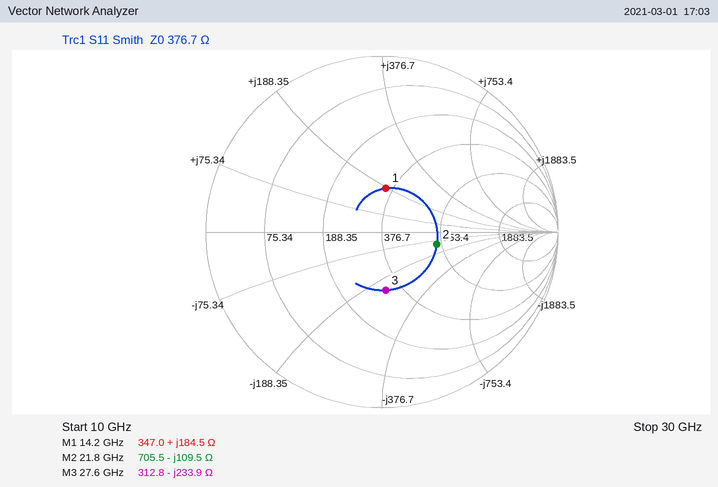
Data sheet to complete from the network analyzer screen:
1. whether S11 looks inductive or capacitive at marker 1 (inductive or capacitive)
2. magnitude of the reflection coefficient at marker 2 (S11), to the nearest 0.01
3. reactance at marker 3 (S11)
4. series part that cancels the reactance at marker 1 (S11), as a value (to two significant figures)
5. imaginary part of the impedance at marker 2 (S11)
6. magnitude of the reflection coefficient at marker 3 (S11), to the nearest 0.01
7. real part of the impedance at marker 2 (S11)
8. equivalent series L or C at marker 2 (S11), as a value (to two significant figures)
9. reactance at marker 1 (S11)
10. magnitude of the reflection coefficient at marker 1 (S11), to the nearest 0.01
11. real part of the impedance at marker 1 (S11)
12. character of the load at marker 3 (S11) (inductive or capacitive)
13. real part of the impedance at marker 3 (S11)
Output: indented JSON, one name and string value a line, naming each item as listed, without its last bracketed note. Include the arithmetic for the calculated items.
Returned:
{
  "whether S11 looks inductive or capacitive at marker 1": "inductive",
  "magnitude of the reflection coefficient at marker 2 (S11), to the nearest 0.01": "0.32",
  "reactance at marker 3": "-233.9 Ω",
  "series part that cancels the reactance at marker 1 (S11), as a value": "C = 1/(2π × 14.2 GHz × 184.5 Ω) ≈ 61 fF",
  "imaginary part of the impedance at marker 2": "-109.5 Ω",
  "magnitude of the reflection coefficient at marker 3 (S11), to the nearest 0.01": "0.33",
  "real part of the impedance at marker 2": "705.5 Ω",
  "equivalent series L or C at marker 2 (S11), as a value": "C = 1/(2π × 21.8 GHz × 109.5 Ω) ≈ 67 fF",
  "reactance at marker 1": "+184.5 Ω",
  "magnitude of the reflection coefficient at marker 1 (S11), to the nearest 0.01": "0.25",
  "real part of the impedance at marker 1": "347.0 Ω",
  "character of the load at marker 3 (S11)": "capacitive",
  "real part of the impedance at marker 3": "312.8 Ω"
}
